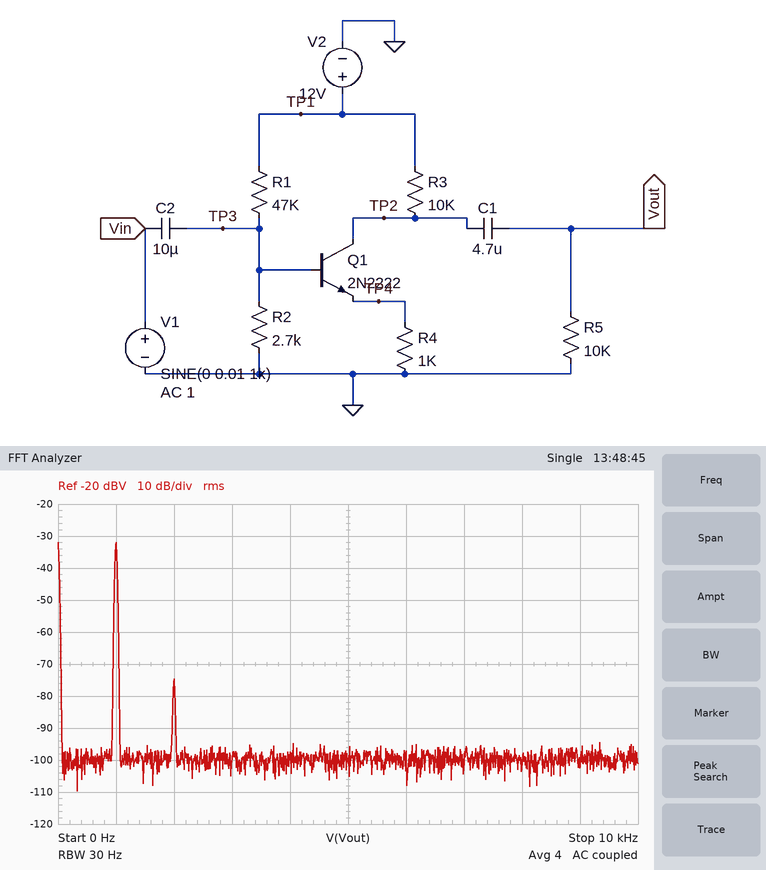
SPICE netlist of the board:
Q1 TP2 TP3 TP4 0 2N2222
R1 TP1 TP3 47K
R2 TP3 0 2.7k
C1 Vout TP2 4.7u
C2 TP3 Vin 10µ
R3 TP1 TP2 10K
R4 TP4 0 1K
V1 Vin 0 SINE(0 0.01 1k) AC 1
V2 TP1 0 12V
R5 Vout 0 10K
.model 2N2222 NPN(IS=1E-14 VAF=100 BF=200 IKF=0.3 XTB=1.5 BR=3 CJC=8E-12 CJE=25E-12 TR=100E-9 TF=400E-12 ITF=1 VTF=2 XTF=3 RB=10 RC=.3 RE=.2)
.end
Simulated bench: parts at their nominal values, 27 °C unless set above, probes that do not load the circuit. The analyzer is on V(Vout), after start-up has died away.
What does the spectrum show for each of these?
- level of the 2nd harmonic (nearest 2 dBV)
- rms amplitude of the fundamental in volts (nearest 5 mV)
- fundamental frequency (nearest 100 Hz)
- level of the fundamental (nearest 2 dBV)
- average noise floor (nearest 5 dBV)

-74 dBV
25 mV
1.0 kHz
-32 dBV
-100 dBV
